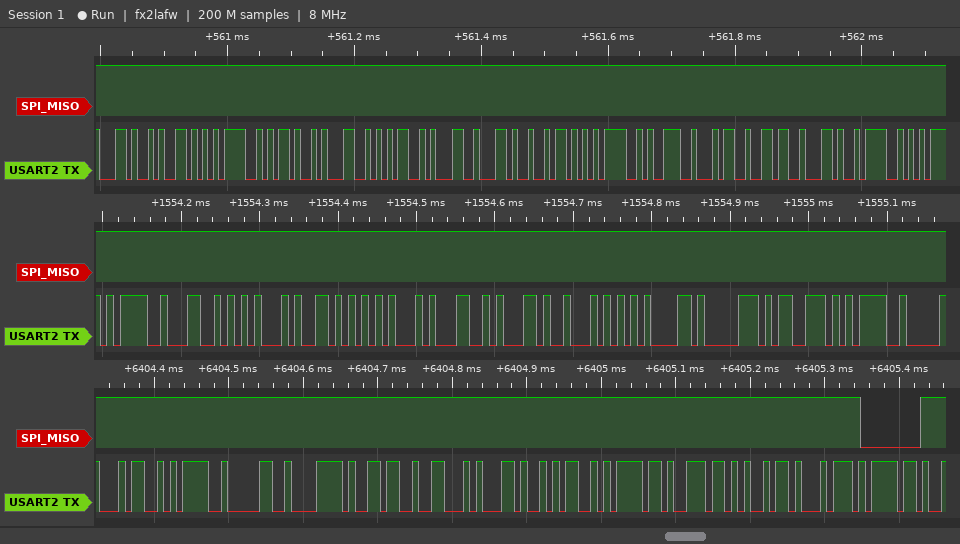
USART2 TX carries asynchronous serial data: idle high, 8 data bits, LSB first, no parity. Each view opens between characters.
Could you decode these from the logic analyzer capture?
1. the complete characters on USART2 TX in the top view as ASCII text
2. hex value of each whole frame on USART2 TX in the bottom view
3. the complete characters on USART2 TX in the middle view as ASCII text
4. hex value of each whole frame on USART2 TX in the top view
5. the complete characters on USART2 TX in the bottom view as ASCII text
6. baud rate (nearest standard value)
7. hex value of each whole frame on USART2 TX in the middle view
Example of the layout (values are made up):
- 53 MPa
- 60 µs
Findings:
- ",Y=-151,Z=946,O"
- 34, 3D, 30, 78, 36, 46, 2C, 4D, 6F, 6E, 69, 74, 6F
- "=LEVEL,Taps="
- 2C, 59, 3D, 2D, 31, 35, 31, 2C, 5A, 3D, 39, 34, 36, 2C, 4F
- "4=0x6F,Monito"
- 115200 baud
- 3D, 4C, 45, 56, 45, 4C, 2C, 54, 61, 70, 73, 3D
